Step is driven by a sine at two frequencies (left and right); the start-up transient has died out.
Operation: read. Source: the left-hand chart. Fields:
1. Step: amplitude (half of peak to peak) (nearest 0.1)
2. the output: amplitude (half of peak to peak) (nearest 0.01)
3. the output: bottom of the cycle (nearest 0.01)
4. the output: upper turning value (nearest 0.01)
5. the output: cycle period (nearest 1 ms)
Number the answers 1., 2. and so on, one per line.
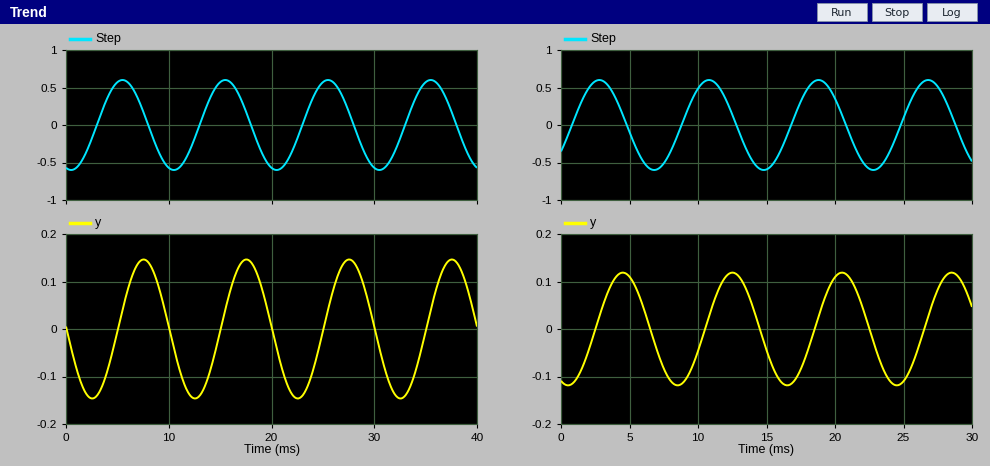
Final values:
1. 0.6
2. 0.15
3. -0.15
4. 0.15
5. 10 ms
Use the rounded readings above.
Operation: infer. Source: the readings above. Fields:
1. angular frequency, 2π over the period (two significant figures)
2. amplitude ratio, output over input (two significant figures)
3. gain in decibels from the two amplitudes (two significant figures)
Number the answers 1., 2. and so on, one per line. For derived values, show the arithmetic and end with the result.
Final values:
1. 2π / 10 = 0.63 rad/ms
2. 0.15 / 0.6 = 0.25
3. 20 log10(0.15 / 0.6) = -12 dB
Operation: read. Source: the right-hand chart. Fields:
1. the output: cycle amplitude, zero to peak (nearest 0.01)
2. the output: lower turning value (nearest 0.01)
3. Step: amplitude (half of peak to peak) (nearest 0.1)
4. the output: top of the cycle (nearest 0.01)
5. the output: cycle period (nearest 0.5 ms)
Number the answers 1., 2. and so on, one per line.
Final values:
1. 0.12
2. -0.12
3. 0.6
4. 0.12
5. 8.0 ms
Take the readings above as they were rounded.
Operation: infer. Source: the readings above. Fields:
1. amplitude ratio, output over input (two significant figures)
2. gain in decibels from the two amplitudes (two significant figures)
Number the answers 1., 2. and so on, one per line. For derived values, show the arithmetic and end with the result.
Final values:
1. 0.12 / 0.6 = 0.20
2. 20 log10(0.12 / 0.6) = -14 dB
